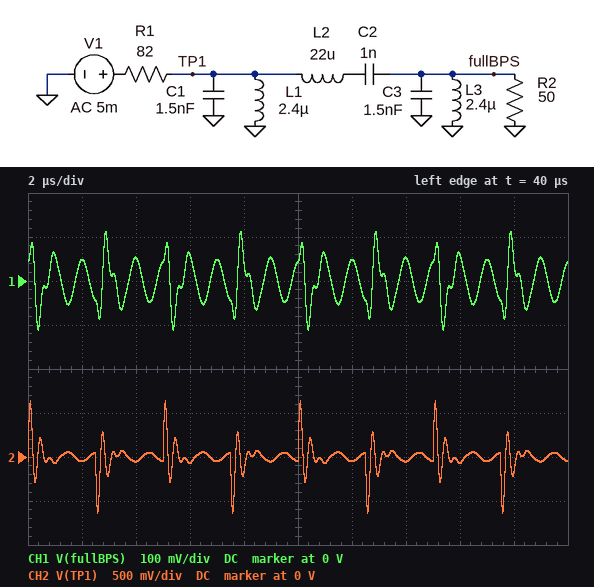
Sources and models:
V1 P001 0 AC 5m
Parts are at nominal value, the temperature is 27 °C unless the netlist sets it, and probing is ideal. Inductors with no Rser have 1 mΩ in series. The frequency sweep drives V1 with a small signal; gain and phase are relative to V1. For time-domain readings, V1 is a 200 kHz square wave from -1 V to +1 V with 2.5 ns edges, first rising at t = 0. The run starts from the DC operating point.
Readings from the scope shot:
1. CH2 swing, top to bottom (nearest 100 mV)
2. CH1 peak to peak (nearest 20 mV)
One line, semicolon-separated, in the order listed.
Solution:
1.3 V; 220 mV
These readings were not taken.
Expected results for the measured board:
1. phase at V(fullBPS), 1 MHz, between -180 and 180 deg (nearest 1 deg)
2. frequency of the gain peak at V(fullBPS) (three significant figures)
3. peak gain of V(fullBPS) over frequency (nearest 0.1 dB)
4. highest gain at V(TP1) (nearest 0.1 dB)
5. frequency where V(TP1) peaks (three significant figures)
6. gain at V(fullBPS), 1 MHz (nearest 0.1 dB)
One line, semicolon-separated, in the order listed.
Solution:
97 deg; 966 kHz; -8.4 dB; -0.3 dB; 2.83 MHz; -12.5 dB
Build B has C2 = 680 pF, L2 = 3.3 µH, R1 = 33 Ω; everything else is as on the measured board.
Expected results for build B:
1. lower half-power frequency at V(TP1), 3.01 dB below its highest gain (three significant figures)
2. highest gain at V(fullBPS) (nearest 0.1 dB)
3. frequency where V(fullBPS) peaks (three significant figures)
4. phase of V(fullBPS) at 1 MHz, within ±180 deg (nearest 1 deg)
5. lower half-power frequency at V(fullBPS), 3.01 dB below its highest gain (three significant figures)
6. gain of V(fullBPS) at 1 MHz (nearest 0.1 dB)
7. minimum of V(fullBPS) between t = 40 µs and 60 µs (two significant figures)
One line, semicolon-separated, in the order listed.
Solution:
1.17 MHz; -4.2 dB; 4.47 MHz; -141 deg; 1.83 MHz; -27.5 dB; -450 mV
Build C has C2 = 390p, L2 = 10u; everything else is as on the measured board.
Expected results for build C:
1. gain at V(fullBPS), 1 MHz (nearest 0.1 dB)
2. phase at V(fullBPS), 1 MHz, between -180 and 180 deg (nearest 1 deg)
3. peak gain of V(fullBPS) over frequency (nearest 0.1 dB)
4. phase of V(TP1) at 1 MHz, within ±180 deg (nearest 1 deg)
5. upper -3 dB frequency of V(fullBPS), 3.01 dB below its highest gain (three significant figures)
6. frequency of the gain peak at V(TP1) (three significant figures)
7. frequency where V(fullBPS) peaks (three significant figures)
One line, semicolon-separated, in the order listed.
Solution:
-39.1 dB; -123 deg; -8.2 dB; 77 deg; 3.69 MHz; 3.62 MHz; 2.09 MHz
